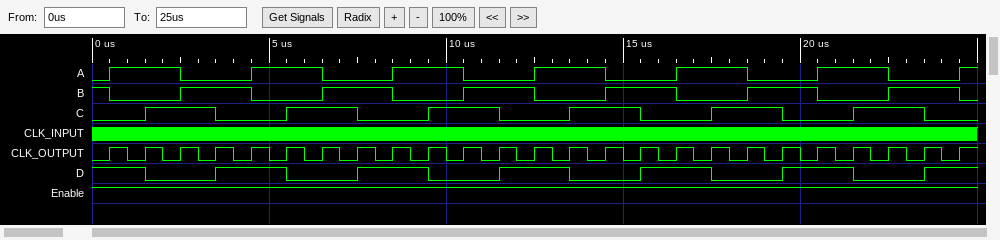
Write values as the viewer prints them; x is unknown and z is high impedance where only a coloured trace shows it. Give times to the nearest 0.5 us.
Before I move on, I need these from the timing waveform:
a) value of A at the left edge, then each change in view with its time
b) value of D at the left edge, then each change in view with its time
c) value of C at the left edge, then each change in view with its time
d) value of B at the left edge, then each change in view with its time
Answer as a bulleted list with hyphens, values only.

- 0, 1 at 0.5 us, 0 at 2.5 us, 1 at 4.5 us, 0 at 6.5 us, 1 at 8.5 us, 0 at 10.5 us, 1 at 12.5 us, 0 at 14.5 us, 1 at 16.5 us, 0 at 18.5 us, 1 at 20.5 us, 0 at 22.5 us, 1 at 24.5 us
- 1, 0 at 1.5 us, 1 at 3.5 us, 0 at 5.5 us, 1 at 7.5 us, 0 at 9.5 us, 1 at 11.5 us, 0 at 13.5 us, 1 at 15.5 us, 0 at 17.5 us, 1 at 19.5 us, 0 at 21.5 us, 1 at 23.5 us
- 0, 1 at 1.5 us, 0 at 3.5 us, 1 at 5.5 us, 0 at 7.5 us, 1 at 9.5 us, 0 at 11.5 us, 1 at 13.5 us, 0 at 15.5 us, 1 at 17.5 us, 0 at 19.5 us, 1 at 21.5 us, 0 at 23.5 us
- 1, 0 at 0.5 us, 1 at 2.5 us, 0 at 4.5 us, 1 at 6.5 us, 0 at 8.5 us, 1 at 10.5 us, 0 at 12.5 us, 1 at 14.5 us, 0 at 16.5 us, 1 at 18.5 us, 0 at 20.5 us, 1 at 22.5 us, 0 at 24.5 us
